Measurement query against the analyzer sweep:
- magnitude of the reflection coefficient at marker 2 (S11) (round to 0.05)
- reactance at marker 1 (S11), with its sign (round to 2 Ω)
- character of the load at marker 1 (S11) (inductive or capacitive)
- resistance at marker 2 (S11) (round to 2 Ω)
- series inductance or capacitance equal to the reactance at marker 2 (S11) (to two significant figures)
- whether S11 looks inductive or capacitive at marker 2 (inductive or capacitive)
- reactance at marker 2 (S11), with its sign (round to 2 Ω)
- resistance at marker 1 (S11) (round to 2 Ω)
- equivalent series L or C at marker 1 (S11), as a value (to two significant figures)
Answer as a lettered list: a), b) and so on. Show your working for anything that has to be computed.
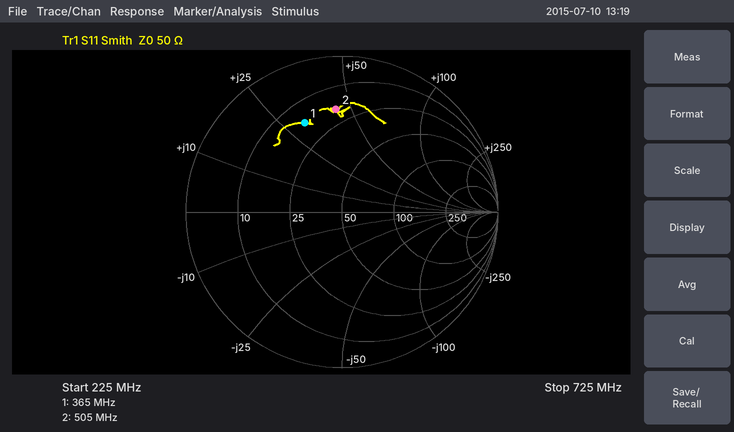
a) 0.65
b) +30 Ω
c) inductive
d) 18 Ω
e) L = 44 Ω/(2π × 505 MHz) ≈ 14 nH
f) inductive
g) +44 Ω
h) 16 Ω
i) L = 30 Ω/(2π × 365 MHz) ≈ 13 nH
